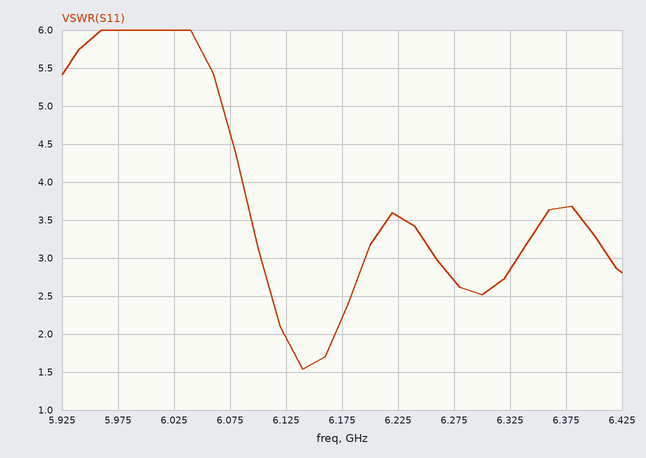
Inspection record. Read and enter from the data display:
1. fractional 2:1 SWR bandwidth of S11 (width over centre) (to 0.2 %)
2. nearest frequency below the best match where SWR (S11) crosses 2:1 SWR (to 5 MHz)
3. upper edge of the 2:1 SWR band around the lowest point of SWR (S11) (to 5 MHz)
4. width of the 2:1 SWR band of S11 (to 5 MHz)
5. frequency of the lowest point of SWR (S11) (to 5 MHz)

0.8 %
6.125 GHz
6.170 GHz
45 MHz
6.140 GHz
